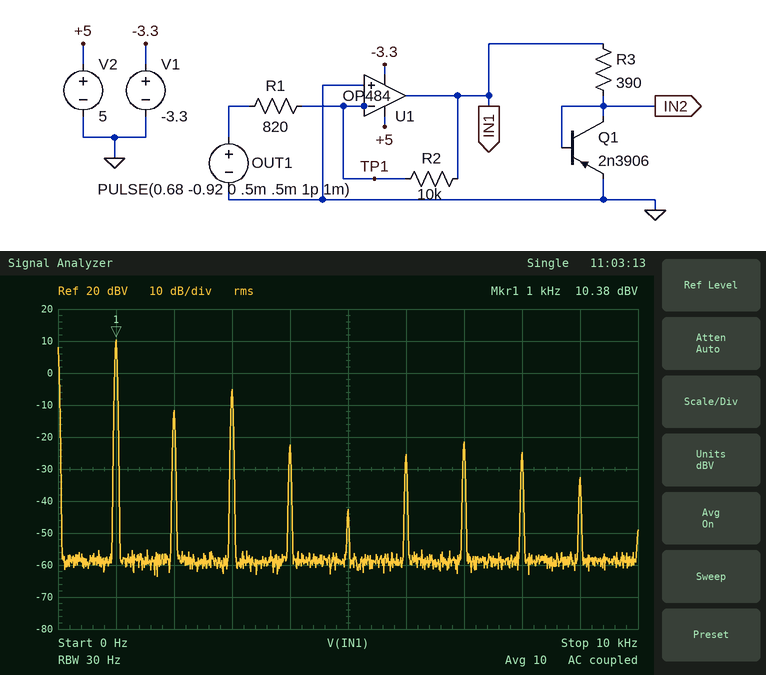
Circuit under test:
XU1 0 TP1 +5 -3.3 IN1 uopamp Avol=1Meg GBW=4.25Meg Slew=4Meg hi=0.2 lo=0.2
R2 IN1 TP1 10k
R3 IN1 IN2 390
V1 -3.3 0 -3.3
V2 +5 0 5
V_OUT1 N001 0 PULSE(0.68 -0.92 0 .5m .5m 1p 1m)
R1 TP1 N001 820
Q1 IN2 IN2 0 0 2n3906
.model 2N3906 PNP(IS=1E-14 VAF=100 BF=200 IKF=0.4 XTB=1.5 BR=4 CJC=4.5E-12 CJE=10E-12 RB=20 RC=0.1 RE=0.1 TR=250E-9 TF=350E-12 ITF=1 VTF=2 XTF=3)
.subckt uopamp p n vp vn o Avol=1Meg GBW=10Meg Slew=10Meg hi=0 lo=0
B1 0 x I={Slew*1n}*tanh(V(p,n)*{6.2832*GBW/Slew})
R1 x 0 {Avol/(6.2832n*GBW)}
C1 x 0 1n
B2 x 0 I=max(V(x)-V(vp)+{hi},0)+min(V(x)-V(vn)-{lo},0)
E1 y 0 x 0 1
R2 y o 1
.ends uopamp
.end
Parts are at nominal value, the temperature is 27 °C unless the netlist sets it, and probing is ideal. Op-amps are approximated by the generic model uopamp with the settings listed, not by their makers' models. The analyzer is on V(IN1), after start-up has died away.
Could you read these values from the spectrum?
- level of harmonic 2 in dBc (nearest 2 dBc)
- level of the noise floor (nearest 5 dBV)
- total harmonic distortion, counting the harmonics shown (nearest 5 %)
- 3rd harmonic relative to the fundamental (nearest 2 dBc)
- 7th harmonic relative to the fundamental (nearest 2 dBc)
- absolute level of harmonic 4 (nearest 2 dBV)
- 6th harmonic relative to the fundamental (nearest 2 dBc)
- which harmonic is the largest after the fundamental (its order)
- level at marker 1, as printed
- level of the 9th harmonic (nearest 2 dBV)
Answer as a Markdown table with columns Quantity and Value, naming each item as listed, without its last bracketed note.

| Quantity | Value |
|---|---|
| level of harmonic 2 in dBc | -22 dBc |
| level of the noise floor | -60 dBV |
| total harmonic distortion, counting the harmonics shown | 20 % |
| 3rd harmonic relative to the fundamental | -16 dBc |
| 7th harmonic relative to the fundamental | -32 dBc |
| absolute level of harmonic 4 | -22 dBV |
| 6th harmonic relative to the fundamental | -36 dBc |
| which harmonic is the largest after the fundamental | 3 |
| level at marker 1, as printed | 10.38 dBV |
| level of the 9th harmonic | -32 dBV |
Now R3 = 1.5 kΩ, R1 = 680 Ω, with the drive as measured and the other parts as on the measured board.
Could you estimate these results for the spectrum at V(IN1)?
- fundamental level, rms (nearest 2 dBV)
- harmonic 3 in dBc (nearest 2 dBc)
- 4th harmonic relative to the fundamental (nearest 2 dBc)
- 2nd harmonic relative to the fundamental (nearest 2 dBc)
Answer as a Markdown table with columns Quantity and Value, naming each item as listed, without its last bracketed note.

| Quantity | Value |
|---|---|
| fundamental level, rms | 10 dBV |
| harmonic 3 in dBc | -14 dBc |
| 4th harmonic relative to the fundamental | -26 dBc |
| 2nd harmonic relative to the fundamental | -20 dBc |
